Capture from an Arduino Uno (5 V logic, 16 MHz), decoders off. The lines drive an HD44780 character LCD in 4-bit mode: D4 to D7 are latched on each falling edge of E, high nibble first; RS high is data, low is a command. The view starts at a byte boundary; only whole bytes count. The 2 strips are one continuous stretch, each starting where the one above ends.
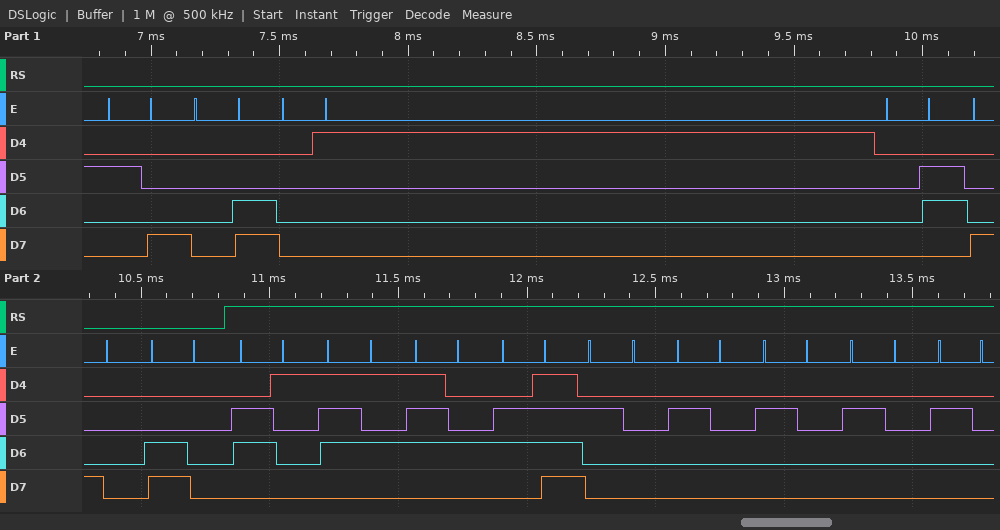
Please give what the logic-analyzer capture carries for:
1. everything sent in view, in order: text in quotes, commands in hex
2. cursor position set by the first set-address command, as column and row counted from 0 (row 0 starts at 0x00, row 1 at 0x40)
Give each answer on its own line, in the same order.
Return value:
0x28 0x0C 0x01 0x06 0x80 0xC0 "auto     "
column 0, row 0
